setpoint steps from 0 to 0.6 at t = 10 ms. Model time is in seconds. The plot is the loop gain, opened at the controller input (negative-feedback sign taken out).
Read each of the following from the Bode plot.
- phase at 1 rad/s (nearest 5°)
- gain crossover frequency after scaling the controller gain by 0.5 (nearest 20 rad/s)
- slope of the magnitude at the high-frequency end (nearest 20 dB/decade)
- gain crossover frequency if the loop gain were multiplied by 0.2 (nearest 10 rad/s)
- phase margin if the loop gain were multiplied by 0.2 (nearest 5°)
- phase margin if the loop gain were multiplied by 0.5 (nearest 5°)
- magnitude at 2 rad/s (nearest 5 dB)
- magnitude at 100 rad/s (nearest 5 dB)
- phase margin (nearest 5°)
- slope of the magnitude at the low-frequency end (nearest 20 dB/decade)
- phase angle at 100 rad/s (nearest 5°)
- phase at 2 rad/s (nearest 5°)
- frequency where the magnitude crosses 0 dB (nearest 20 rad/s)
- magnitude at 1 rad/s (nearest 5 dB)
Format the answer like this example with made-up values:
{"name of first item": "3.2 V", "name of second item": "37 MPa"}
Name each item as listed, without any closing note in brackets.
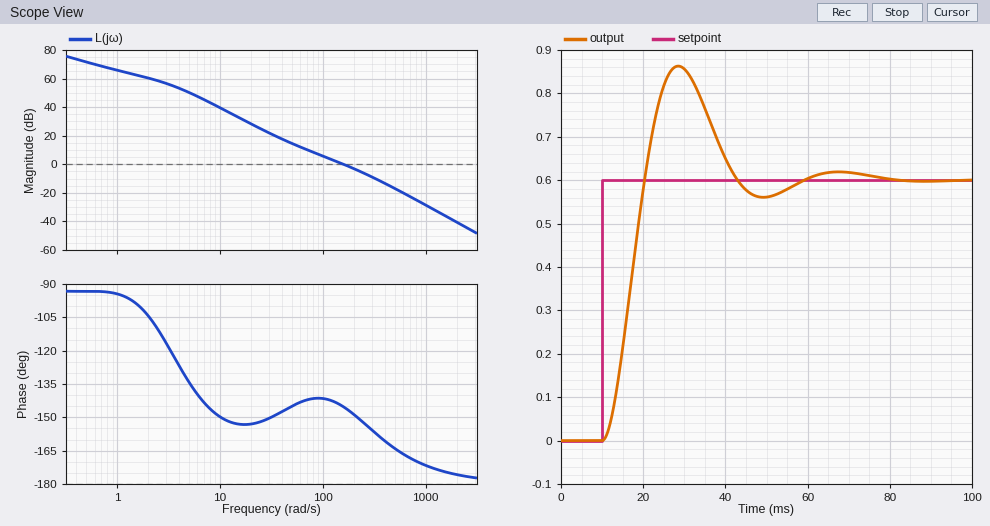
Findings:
{"phase at 1 rad/s": "-95°", "gain crossover frequency after scaling the controller gain by 0.5": "100 rad/s", "slope of the magnitude at the high-frequency end": "-40 dB/decade", "gain crossover frequency if the loop gain were multiplied by 0.2": "50 rad/s", "phase margin if the loop gain were multiplied by 0.2": "35°", "phase margin if the loop gain were multiplied by 0.5": "40°", "magnitude at 2 rad/s": "60 dB", "magnitude at 100 rad/s": "5 dB", "phase margin": "35°", "slope of the magnitude at the low-frequency end": "-20 dB/decade", "phase angle at 100 rad/s": "-140°", "phase at 2 rad/s": "-105°", "frequency where the magnitude crosses 0 dB": "160 rad/s", "magnitude at 1 rad/s": "65 dB"}
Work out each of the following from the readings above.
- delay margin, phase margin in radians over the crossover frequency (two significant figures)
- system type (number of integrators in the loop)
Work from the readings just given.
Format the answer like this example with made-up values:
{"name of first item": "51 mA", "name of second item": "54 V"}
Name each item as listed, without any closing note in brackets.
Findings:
{"delay margin, phase margin in radians over the crossover frequency": "0.0038 s", "system type": "1"}
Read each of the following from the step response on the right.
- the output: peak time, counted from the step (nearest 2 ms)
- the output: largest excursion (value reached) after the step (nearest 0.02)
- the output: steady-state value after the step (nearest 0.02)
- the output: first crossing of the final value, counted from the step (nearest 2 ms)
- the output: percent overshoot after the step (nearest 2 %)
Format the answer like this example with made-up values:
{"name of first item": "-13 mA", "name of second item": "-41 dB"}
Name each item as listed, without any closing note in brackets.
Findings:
{"the output: peak time, counted from the step": "18 ms", "the output: largest excursion (value reached) after the step": "0.86", "the output: steady-state value after the step": "0.60", "the output: first crossing of the final value, counted from the step": "10 ms", "the output: percent overshoot after the step": "44 %"}
